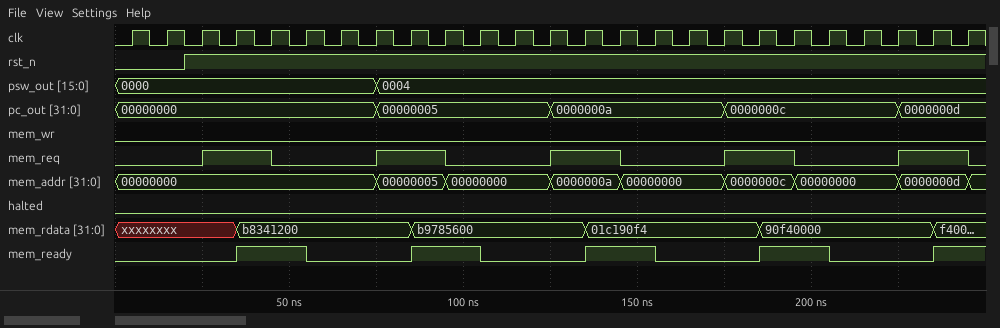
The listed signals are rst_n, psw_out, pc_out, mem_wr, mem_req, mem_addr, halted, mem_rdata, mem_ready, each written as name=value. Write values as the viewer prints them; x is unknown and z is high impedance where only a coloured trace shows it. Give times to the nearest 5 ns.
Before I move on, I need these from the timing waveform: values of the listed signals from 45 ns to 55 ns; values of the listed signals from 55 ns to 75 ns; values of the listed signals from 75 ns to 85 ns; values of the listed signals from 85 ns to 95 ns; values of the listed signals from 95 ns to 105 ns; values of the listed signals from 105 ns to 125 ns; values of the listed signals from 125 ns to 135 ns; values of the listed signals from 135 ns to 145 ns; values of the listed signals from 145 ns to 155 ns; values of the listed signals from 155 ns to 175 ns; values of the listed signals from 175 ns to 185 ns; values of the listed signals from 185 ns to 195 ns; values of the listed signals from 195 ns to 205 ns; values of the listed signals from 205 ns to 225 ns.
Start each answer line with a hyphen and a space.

- rst_n=1, psw_out=0000, pc_out=00000000, mem_wr=0, mem_req=0, mem_addr=00000000, halted=0, mem_rdata=b8341200, mem_ready=1
- rst_n=1, psw_out=0000, pc_out=00000000, mem_wr=0, mem_req=0, mem_addr=00000000, halted=0, mem_rdata=b8341200, mem_ready=0
- rst_n=1, psw_out=0004, pc_out=00000005, mem_wr=0, mem_req=1, mem_addr=00000005, halted=0, mem_rdata=b8341200, mem_ready=0
- rst_n=1, psw_out=0004, pc_out=00000005, mem_wr=0, mem_req=1, mem_addr=00000005, halted=0, mem_rdata=b9785600, mem_ready=1
- rst_n=1, psw_out=0004, pc_out=00000005, mem_wr=0, mem_req=0, mem_addr=00000000, halted=0, mem_rdata=b9785600, mem_ready=1
- rst_n=1, psw_out=0004, pc_out=00000005, mem_wr=0, mem_req=0, mem_addr=00000000, halted=0, mem_rdata=b9785600, mem_ready=0
- rst_n=1, psw_out=0004, pc_out=0000000a, mem_wr=0, mem_req=1, mem_addr=0000000a, halted=0, mem_rdata=b9785600, mem_ready=0
- rst_n=1, psw_out=0004, pc_out=0000000a, mem_wr=0, mem_req=1, mem_addr=0000000a, halted=0, mem_rdata=01c190f4, mem_ready=1
- rst_n=1, psw_out=0004, pc_out=0000000a, mem_wr=0, mem_req=0, mem_addr=00000000, halted=0, mem_rdata=01c190f4, mem_ready=1
- rst_n=1, psw_out=0004, pc_out=0000000a, mem_wr=0, mem_req=0, mem_addr=00000000, halted=0, mem_rdata=01c190f4, mem_ready=0
- rst_n=1, psw_out=0004, pc_out=0000000c, mem_wr=0, mem_req=1, mem_addr=0000000c, halted=0, mem_rdata=01c190f4, mem_ready=0
- rst_n=1, psw_out=0004, pc_out=0000000c, mem_wr=0, mem_req=1, mem_addr=0000000c, halted=0, mem_rdata=90f40000, mem_ready=1
- rst_n=1, psw_out=0004, pc_out=0000000c, mem_wr=0, mem_req=0, mem_addr=00000000, halted=0, mem_rdata=90f40000, mem_ready=1
- rst_n=1, psw_out=0004, pc_out=0000000c, mem_wr=0, mem_req=0, mem_addr=00000000, halted=0, mem_rdata=90f40000, mem_ready=0
